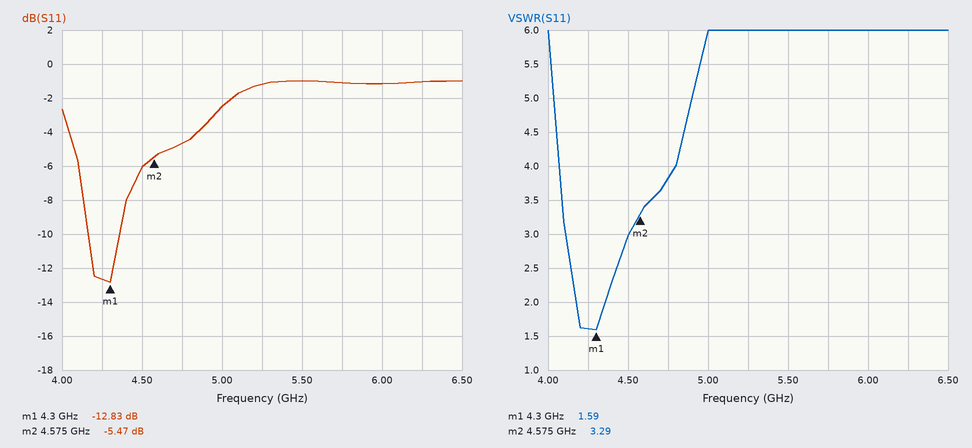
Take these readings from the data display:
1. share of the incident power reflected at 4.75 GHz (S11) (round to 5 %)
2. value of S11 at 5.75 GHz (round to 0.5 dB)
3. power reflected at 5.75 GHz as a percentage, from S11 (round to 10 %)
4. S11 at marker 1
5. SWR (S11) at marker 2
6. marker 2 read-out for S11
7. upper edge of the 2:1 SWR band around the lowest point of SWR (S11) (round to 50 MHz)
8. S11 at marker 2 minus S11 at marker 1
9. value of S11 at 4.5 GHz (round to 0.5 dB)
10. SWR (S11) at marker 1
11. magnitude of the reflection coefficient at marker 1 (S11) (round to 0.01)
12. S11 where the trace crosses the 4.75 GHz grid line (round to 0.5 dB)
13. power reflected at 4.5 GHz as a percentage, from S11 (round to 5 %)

35 %
-1.0 dB
80 %
-12.83 dB
3.29
-5.47 dB
4.35 GHz
7.36 dB
-6.0 dB
1.59
0.23
-4.5 dB
25 %
